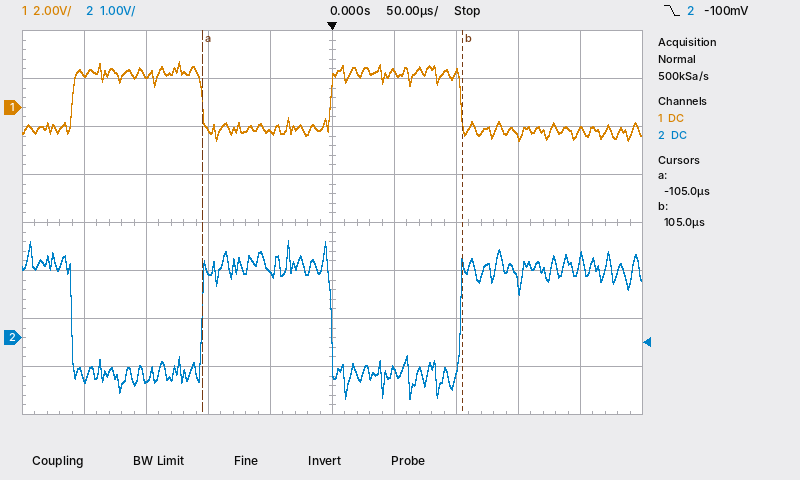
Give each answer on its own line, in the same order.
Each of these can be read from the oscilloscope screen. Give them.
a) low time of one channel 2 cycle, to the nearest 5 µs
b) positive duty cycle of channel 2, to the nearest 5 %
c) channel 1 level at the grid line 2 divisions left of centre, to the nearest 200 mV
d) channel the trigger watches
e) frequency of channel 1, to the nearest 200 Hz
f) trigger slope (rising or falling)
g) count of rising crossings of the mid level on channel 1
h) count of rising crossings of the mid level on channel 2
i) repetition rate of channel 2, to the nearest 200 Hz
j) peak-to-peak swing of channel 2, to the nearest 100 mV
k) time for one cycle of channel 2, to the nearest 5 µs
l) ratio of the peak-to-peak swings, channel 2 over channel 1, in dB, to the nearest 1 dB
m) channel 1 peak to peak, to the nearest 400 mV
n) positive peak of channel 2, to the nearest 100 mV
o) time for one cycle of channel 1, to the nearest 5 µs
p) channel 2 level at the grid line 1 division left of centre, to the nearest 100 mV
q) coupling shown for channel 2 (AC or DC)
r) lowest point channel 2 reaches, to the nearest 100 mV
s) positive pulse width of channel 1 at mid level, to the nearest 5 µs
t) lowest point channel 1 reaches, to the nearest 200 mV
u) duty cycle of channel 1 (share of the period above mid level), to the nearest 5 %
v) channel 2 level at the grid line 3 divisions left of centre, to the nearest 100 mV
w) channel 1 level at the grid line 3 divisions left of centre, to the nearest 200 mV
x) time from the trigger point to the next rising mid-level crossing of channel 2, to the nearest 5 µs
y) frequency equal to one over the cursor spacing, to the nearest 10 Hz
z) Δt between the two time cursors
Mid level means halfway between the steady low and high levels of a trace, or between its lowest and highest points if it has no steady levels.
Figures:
105 µs
50 %
-1.0 V
channel 2
4.8 kHz
falling
2
2
4.8 kHz
3.3 V
210 µs
0 dB
3.2 V
2.0 V
210 µs
1.4 V
DC
-1.3 V
105 µs
-1.4 V
50 %
-800 mV
1.4 V
105 µs
4.76 kHz
210 µs
